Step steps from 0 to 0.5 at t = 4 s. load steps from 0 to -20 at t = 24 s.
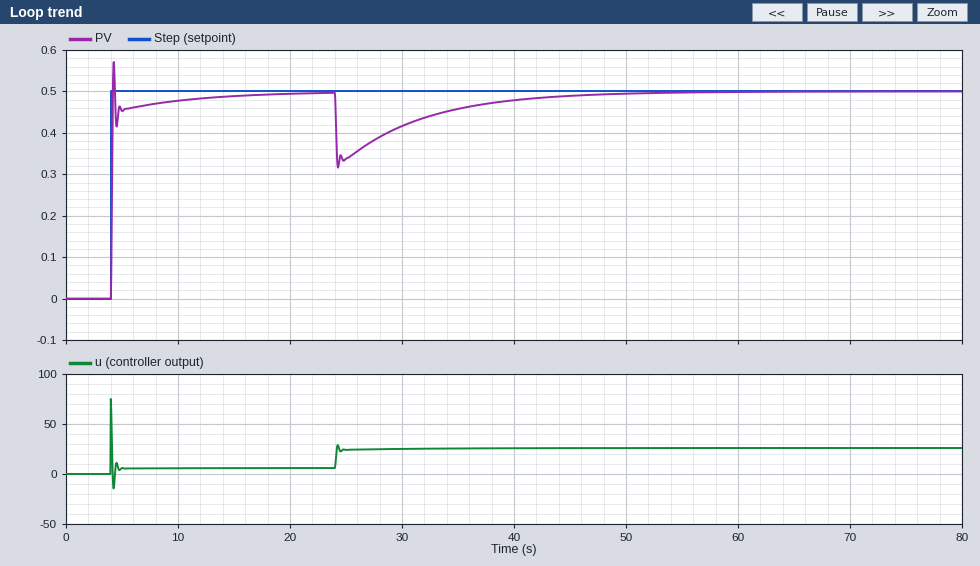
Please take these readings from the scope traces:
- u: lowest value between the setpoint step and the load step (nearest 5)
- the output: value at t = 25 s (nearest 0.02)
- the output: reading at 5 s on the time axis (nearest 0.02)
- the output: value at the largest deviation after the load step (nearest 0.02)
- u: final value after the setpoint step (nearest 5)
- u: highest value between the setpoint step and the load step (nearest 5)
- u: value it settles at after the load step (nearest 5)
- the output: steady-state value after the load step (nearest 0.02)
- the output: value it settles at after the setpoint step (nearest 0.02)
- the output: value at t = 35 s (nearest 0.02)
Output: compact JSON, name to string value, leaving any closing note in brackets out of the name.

{"u: lowest value between the setpoint step and the load step": "-15", "the output: value at t = 25 s": "0.34", "the output: reading at 5 s on the time axis": "0.46", "the output: value at the largest deviation after the load step": "0.32", "u: final value after the setpoint step": "5", "u: highest value between the setpoint step and the load step": "75", "u: value it settles at after the load step": "25", "the output: steady-state value after the load step": "0.50", "the output: value it settles at after the setpoint step": "0.50", "the output: value at t = 35 s": "0.46"}
